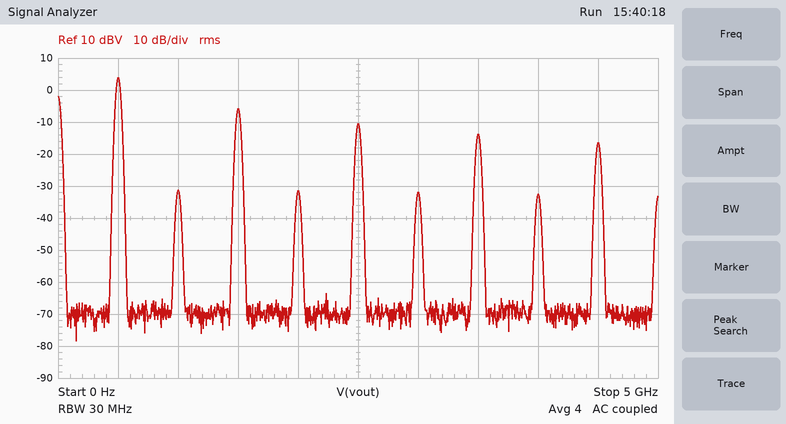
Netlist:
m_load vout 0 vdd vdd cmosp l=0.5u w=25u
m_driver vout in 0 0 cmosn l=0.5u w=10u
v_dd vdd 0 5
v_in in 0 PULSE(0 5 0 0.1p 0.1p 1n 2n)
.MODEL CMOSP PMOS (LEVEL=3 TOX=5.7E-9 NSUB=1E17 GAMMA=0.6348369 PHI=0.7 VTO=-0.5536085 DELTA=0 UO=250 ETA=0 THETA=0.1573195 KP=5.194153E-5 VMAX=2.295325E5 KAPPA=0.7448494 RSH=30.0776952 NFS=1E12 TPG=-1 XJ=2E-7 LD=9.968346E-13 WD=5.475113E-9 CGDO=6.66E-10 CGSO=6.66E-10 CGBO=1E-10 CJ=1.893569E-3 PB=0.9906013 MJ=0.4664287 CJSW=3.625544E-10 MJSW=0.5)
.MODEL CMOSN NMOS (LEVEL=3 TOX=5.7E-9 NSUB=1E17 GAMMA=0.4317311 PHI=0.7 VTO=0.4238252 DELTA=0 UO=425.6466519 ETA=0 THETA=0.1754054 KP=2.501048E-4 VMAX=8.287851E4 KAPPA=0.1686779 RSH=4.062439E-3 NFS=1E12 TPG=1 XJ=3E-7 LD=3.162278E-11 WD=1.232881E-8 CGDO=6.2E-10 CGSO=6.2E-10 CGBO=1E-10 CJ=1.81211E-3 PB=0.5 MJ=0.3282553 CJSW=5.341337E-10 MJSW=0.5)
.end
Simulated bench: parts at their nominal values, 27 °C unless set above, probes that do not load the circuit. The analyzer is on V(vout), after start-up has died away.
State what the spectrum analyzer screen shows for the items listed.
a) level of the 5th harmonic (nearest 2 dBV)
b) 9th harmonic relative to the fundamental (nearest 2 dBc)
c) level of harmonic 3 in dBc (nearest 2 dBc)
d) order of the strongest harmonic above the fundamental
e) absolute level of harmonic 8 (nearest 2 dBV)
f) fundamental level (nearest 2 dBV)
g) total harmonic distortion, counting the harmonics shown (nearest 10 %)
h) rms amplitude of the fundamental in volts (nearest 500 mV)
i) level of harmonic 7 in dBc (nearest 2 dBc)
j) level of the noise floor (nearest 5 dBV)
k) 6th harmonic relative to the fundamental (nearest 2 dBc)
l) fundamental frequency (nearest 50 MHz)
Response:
-10 dBV
-20 dBc
-10 dBc
3
-32 dBV
4 dBV
40 %
1.5 V
-18 dBc
-70 dBV
-36 dBc
500 MHz
